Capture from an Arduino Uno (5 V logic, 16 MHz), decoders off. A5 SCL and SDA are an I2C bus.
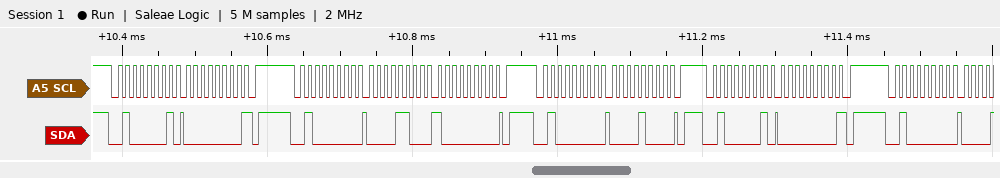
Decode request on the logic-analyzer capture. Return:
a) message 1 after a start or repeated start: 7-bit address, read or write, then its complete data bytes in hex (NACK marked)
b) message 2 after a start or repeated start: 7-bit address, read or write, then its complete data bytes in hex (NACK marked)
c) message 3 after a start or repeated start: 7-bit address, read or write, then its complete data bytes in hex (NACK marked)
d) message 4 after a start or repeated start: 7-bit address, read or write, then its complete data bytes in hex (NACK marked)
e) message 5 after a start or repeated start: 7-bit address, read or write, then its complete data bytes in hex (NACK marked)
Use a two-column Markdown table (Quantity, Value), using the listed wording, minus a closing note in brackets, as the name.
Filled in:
| Quantity | Value |
|---|---|
| message 1 after a start or repeated start: 7-bit address, read or write, then its complete data bytes in hex | 0x20 read: 00 NACK |
| message 2 after a start or repeated start: 7-bit address, read or write, then its complete data bytes in hex | 0x20 write: 0C 80 |
| message 3 after a start or repeated start: 7-bit address, read or write, then its complete data bytes in hex | 0x20 write: 08 |
| message 4 after a start or repeated start: 7-bit address, read or write, then its complete data bytes in hex | 0x20 read: 00 NACK |
| message 5 after a start or repeated start: 7-bit address, read or write, then its complete data bytes in hex | 0x20 write |
